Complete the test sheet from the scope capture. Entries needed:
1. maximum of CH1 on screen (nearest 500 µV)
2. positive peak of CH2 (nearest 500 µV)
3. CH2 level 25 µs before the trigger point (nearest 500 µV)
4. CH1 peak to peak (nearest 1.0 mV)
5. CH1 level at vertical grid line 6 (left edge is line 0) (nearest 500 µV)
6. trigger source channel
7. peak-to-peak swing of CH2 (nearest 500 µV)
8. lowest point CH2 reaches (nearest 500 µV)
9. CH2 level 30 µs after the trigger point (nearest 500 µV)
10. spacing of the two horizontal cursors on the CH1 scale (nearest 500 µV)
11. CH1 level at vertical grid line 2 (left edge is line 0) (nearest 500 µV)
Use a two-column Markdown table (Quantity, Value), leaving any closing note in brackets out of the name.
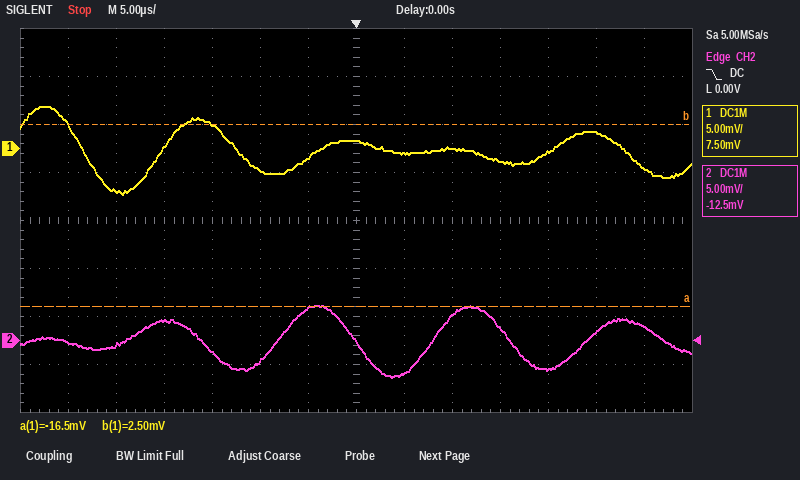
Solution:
| Quantity | Value |
|---|---|
| maximum of CH1 on screen | 4.5 mV |
| positive peak of CH2 | 3.5 mV |
| CH2 level 25 µs before the trigger point | -500 µV |
| CH1 peak to peak | 9.0 mV |
| CH1 level at vertical grid line 6 (left edge is line 0) | -1.0 mV |
| trigger source channel | CH2 |
| peak-to-peak swing of CH2 | 7.5 mV |
| lowest point CH2 reaches | -4.0 mV |
| CH2 level 30 µs after the trigger point | 1.5 mV |
| spacing of the two horizontal cursors on the CH1 scale | 19.0 mV |
| CH1 level at vertical grid line 2 (left edge is line 0) | -4.5 mV |
